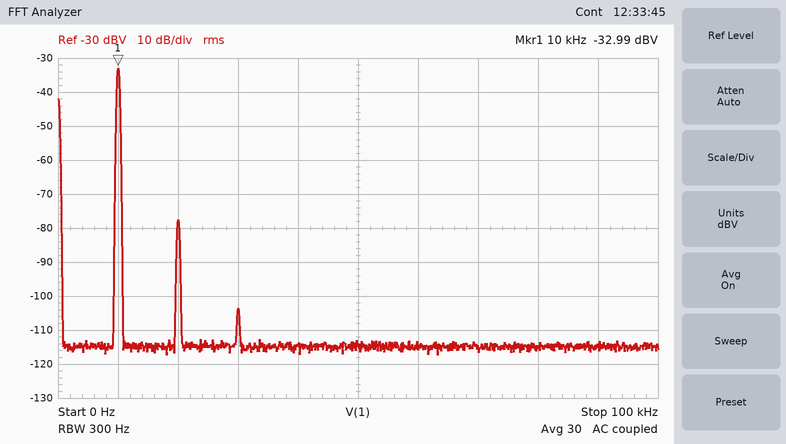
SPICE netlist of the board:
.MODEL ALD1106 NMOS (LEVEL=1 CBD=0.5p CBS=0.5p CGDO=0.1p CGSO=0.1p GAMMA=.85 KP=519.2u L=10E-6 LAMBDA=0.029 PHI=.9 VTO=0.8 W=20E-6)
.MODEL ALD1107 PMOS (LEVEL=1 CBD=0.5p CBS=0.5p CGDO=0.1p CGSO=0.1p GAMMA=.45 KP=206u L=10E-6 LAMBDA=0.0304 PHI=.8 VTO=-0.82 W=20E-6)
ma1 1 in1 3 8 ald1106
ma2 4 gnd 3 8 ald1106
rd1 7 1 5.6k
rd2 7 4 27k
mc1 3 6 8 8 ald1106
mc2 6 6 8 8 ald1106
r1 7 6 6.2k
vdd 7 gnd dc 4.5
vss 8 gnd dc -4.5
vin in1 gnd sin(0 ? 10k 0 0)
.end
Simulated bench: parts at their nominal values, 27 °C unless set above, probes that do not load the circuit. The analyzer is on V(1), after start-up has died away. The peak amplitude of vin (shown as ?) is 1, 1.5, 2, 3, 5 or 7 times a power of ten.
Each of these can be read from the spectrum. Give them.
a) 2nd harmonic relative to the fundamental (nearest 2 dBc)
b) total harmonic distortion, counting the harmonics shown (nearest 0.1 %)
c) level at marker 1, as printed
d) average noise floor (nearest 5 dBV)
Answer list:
-44 dBc
0.6 %
-32.99 dBV
-115 dBV
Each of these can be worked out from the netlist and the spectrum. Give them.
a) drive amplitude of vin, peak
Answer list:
100 mV
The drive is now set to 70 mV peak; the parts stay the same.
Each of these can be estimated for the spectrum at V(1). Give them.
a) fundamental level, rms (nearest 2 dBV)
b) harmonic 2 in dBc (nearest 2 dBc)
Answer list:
-36 dBV
-48 dBc
